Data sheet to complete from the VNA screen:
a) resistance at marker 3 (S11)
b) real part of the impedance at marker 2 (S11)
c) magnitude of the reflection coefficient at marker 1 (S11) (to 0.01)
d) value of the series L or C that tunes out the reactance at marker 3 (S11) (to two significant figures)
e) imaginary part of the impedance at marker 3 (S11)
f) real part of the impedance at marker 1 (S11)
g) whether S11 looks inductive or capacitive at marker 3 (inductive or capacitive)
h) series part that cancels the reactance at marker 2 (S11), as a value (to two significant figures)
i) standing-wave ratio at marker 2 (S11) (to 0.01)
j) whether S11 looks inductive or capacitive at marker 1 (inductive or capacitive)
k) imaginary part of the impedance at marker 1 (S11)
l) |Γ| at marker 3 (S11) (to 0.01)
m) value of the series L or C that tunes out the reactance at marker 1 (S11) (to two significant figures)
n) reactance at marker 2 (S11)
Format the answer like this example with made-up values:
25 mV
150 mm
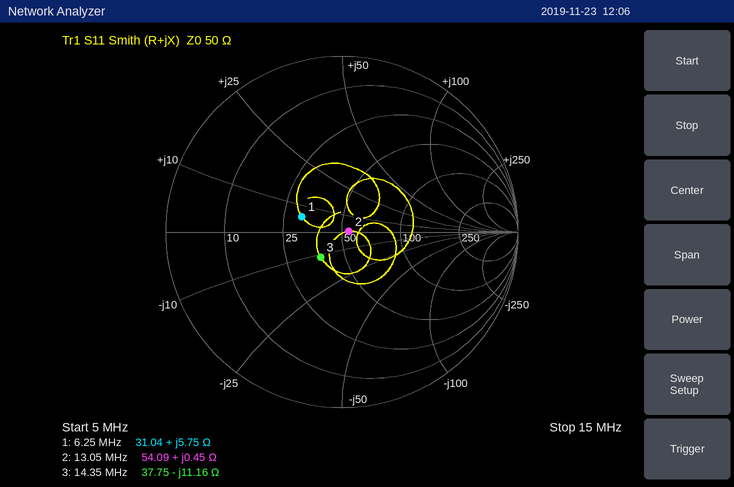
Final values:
37.75 Ω
54.09 Ω
0.24
120 nH
-11.16 Ω
31.04 Ω
capacitive
27 nF
1.08
inductive
+5.75 Ω
0.19
4.4 nF
+0.45 Ω
